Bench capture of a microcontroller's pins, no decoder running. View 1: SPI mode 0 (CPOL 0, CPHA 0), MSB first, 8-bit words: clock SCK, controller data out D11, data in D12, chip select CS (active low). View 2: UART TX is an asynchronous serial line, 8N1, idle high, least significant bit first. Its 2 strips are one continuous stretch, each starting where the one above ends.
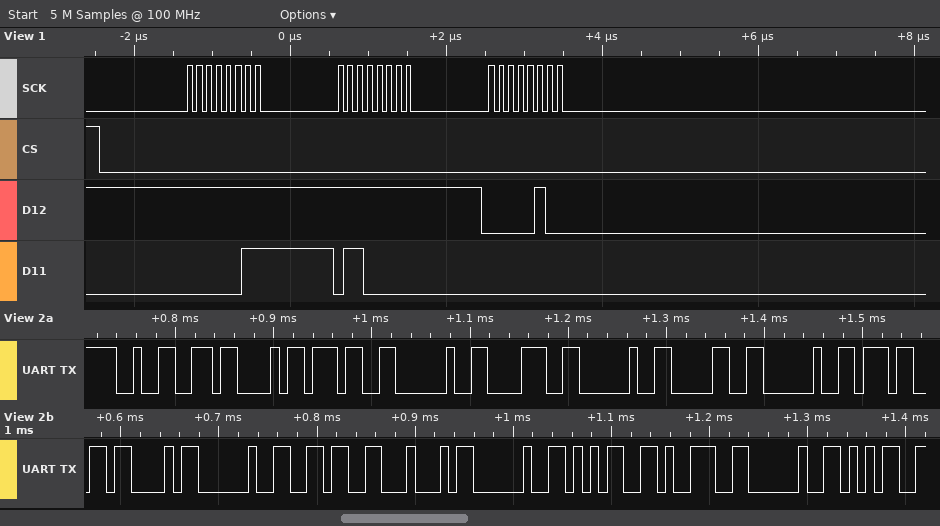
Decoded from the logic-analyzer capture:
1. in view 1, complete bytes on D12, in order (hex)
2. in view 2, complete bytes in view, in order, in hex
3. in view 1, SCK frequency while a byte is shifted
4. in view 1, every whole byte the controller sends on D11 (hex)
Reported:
FF FF 04
0x32 0x43 0x37 0x20 0x38 0x20 0x30 0x20 0x37 0x43 0x20 0x36 0x44 0x20 0x35 0x39 0x20 0x35
8 MHz
03 60 00
